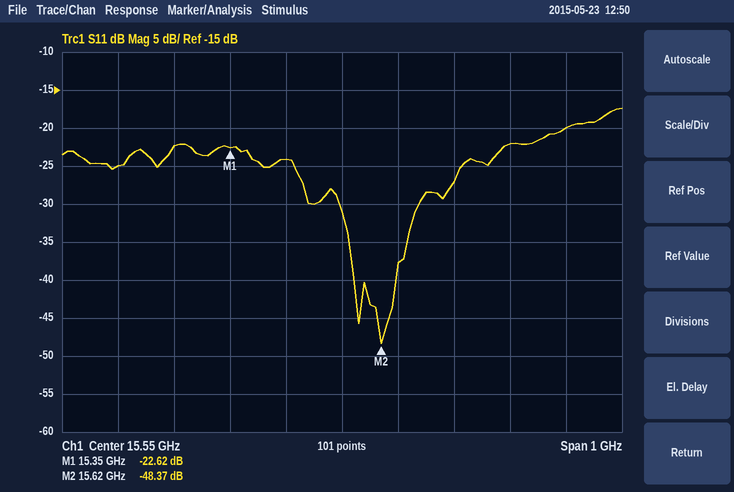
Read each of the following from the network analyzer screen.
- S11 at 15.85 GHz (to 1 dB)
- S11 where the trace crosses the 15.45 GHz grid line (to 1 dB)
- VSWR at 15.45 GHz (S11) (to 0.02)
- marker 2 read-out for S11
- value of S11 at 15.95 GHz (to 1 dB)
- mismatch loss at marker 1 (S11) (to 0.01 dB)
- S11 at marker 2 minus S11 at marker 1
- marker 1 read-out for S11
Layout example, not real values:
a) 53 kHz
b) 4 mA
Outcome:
a) -22 dB
b) -24 dB
c) 1.14
d) -48.37 dB
e) -20 dB
f) 0.02 dB
g) -25.75 dB
h) -22.62 dB
